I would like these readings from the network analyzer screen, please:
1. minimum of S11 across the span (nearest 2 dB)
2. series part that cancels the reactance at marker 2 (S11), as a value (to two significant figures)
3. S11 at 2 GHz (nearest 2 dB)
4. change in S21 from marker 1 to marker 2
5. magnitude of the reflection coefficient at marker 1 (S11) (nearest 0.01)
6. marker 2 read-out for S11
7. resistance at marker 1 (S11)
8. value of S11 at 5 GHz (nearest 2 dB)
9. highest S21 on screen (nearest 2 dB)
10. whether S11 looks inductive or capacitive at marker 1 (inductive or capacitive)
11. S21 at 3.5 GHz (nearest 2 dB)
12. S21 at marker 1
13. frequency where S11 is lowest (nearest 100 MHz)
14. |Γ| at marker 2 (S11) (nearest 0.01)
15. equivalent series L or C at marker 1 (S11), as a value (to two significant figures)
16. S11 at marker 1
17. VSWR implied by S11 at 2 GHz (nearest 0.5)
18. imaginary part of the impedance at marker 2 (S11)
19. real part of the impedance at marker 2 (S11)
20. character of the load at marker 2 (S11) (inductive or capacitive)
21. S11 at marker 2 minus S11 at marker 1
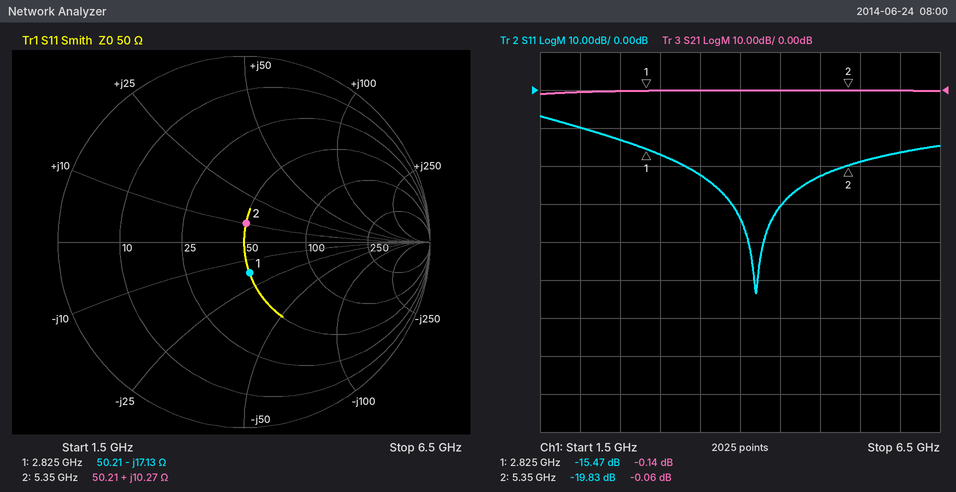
-54 dB
2.9 pF
-10 dB
0.08 dB
0.17
-19.83 dB
50.21 Ω
-22 dB
0 dB
capacitive
0 dB
-0.14 dB
4.2 GHz
0.10
3.3 pF
-15.47 dB
2.0
+10.27 Ω
50.21 Ω
inductive
-4.36 dB
